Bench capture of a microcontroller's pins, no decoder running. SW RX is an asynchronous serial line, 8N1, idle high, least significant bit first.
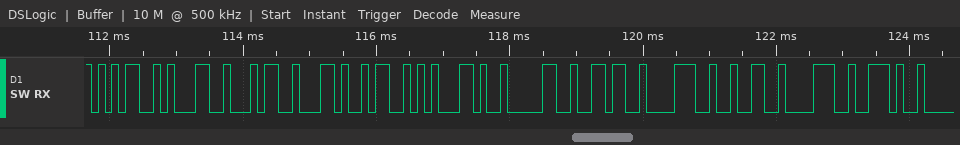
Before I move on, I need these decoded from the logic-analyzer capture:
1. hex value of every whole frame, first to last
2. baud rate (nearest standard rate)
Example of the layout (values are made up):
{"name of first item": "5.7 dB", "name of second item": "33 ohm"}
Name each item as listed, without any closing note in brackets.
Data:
{"hex value of every whole frame, first to last": "0x35 0x31 0x34 0x2C 0x53 0x2C 0x30 0x36 0x38 0x32 0x38 0x2E", "baud rate": "9600 baud"}
